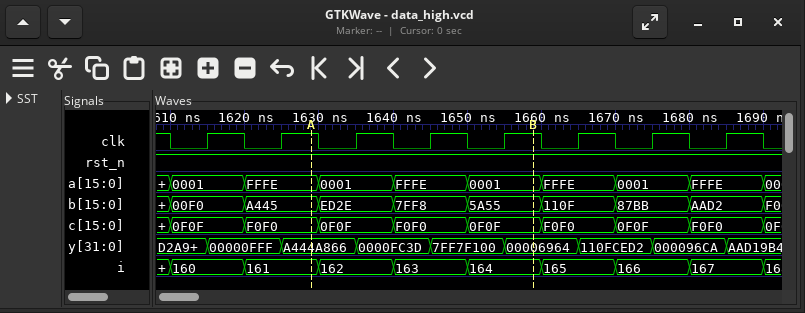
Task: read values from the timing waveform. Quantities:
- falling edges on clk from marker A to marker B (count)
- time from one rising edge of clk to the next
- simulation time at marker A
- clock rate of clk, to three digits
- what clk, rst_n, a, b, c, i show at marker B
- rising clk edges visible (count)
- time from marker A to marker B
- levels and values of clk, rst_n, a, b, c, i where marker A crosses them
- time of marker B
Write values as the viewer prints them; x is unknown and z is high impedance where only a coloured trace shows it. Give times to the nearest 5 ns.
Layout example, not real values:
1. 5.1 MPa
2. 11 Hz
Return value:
1. 3
2. 10 ns
3. 1630 ns
4. 100 MHz
5. clk=1, rst_n=1, a=0001, b=5A55, c=0F0F, i=164
6. 8
7. 30 ns
8. clk=1, rst_n=1, a=FFFE, b=A445, c=F0F0, i=161
9. 1660 ns
